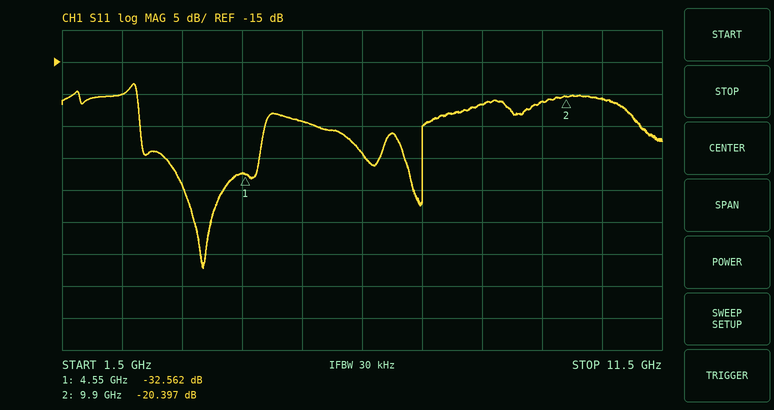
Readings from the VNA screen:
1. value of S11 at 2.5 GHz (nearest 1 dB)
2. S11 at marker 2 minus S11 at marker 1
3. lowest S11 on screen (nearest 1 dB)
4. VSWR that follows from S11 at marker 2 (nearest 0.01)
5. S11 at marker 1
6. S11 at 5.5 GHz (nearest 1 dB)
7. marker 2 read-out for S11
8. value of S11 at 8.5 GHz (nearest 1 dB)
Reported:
-20 dB
12.165 dB
-47 dB
1.21
-32.562 dB
-24 dB
-20.397 dB
-22 dB
